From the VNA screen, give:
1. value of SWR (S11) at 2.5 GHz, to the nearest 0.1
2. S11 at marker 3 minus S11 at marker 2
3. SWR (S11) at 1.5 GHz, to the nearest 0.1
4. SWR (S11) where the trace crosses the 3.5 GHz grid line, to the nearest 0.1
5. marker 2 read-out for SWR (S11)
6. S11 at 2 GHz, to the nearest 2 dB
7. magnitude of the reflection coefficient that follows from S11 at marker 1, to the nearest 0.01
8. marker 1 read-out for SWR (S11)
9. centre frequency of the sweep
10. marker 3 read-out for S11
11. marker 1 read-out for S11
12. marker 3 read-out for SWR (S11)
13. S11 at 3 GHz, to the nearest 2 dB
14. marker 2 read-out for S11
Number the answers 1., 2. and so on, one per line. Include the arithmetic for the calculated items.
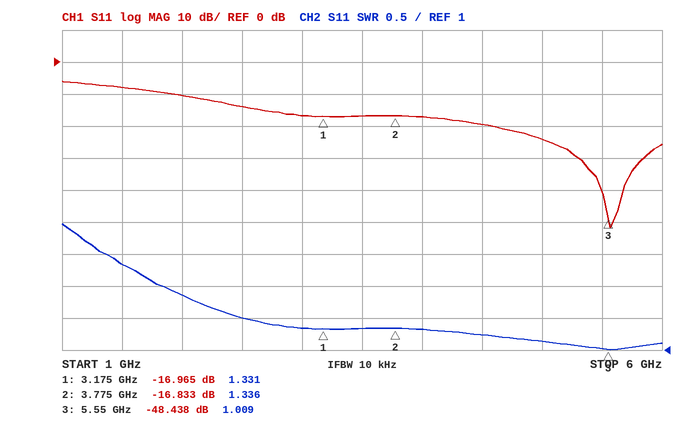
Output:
1. 1.5
2. -48.438 − (-16.833) = -31.605 dB
3. 2.3
4. 1.3
5. 1.336
6. -10 dB
7. 10^(-16.965/20) ≈ 0.14
8. 1.331
9. 3.5 GHz
10. -48.438 dB
11. -16.965 dB
12. 1.009
13. -16 dB
14. -16.833 dB
